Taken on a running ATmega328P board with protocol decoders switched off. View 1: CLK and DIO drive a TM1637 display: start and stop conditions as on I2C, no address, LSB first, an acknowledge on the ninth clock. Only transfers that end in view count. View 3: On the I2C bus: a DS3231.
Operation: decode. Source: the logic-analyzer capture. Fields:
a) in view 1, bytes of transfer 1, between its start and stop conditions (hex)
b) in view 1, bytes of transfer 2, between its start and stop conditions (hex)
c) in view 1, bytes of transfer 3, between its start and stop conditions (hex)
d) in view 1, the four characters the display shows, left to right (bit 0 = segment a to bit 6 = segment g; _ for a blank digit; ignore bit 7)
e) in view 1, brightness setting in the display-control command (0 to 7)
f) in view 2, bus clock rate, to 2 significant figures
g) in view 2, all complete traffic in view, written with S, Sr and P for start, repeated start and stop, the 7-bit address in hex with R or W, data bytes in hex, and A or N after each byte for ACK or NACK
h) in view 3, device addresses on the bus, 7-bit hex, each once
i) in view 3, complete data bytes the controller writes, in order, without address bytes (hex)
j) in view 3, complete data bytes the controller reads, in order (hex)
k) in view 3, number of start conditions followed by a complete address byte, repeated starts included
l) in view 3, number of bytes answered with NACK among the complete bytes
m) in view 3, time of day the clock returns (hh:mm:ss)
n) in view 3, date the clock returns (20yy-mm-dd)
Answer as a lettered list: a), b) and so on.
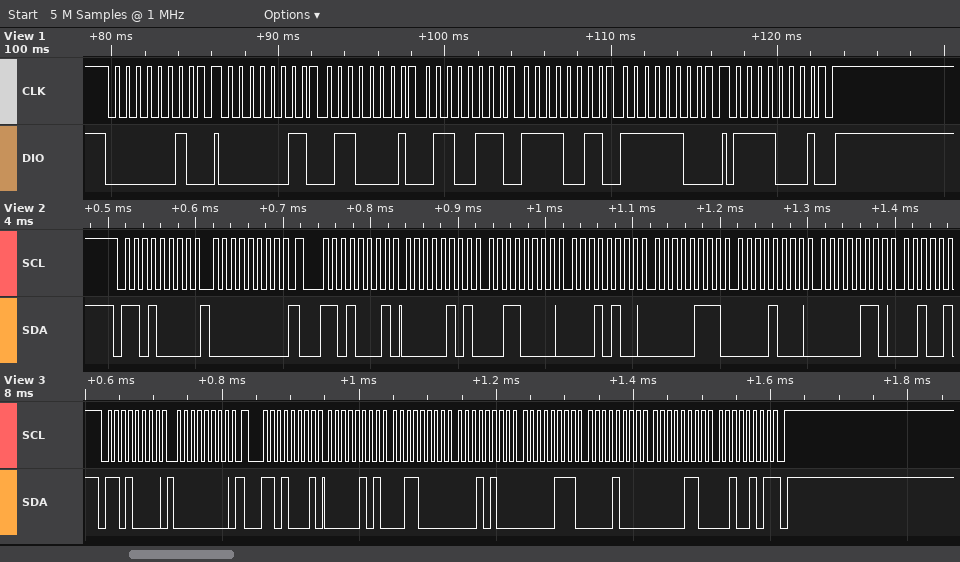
a) 40
b) C0 86 E6 CF 3F
c) 8F
d) 1430
e) 7
f) 100 kHz
g) S 68W A 00 A Sr 68R A 05 A 30 A 14 A 07 A 08 A 06 A
h) 0x68
i) 00
j) 05 30 14 07 08 06 25
k) 2
l) 1
m) 14:30:05
n) 2025-06-08
